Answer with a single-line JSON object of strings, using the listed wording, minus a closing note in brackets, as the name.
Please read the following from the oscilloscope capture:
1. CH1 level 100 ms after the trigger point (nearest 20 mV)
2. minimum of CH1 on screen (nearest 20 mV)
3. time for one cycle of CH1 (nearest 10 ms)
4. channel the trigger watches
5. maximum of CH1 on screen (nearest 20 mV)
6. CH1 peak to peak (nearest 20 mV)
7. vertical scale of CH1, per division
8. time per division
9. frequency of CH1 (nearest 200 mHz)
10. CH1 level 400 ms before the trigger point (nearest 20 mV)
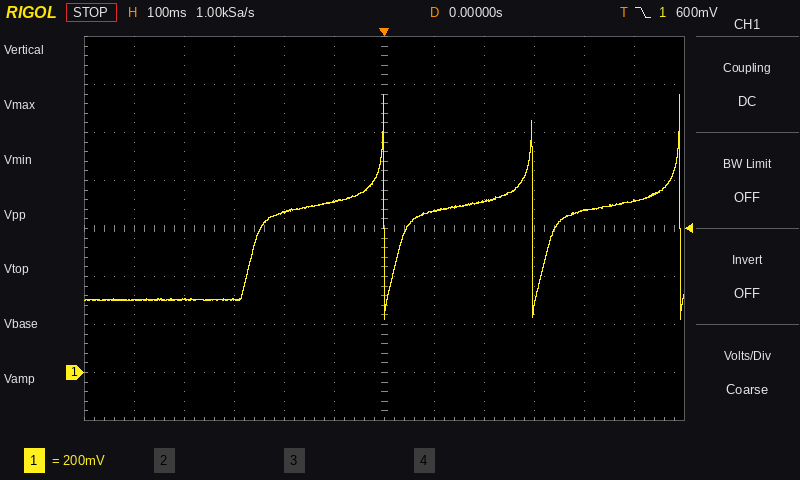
{"CH1 level 100 ms after the trigger point": "680 mV", "minimum of CH1 on screen": "220 mV", "time for one cycle of CH1": "300 ms", "channel the trigger watches": "CH1", "maximum of CH1 on screen": "1.16 V", "CH1 peak to peak": "940 mV", "vertical scale of CH1, per division": "200 mV", "time per division": "100 ms", "frequency of CH1": "3.4 Hz", "CH1 level 400 ms before the trigger point": "300 mV"}
